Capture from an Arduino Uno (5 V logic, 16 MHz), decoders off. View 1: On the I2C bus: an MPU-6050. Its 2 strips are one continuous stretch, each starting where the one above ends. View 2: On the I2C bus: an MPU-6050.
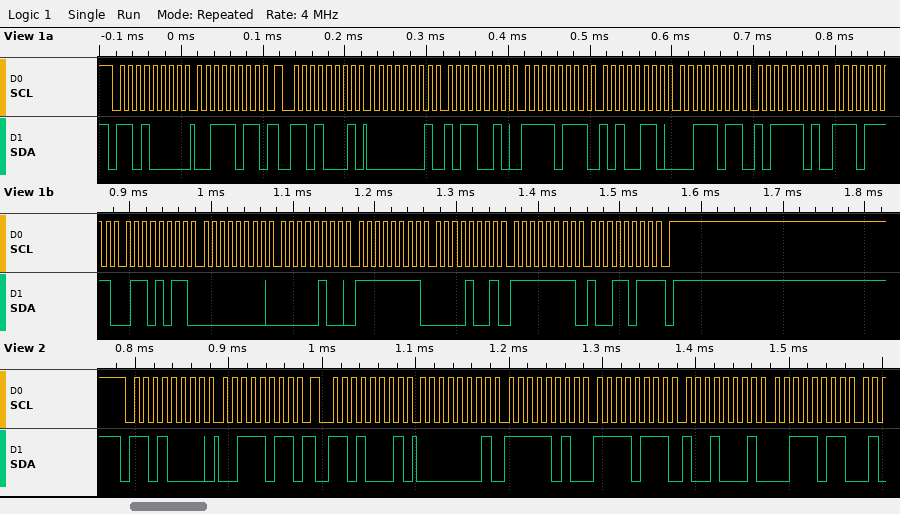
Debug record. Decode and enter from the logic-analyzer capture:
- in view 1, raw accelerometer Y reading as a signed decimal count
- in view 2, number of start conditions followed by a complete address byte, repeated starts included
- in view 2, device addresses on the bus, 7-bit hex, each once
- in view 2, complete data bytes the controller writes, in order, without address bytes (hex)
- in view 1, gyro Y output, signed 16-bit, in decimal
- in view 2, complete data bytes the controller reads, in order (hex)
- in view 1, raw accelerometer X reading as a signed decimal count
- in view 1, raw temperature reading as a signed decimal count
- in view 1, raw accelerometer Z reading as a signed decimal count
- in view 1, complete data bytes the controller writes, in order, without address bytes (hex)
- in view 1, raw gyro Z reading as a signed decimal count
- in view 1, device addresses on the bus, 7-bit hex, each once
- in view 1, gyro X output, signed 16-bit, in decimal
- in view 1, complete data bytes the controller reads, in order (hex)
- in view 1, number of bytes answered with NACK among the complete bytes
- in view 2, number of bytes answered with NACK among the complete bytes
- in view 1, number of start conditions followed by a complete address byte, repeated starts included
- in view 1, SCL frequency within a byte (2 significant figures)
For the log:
-2138
2
0x68
3B
-247
01 FA F7 91 3B
434
-4245
15293
3B
-101
0x68
4
01 B2 F7 A6 3B BD EF 6B 00 04 FF 09 FF 9B
1
0
2
100 kHz
